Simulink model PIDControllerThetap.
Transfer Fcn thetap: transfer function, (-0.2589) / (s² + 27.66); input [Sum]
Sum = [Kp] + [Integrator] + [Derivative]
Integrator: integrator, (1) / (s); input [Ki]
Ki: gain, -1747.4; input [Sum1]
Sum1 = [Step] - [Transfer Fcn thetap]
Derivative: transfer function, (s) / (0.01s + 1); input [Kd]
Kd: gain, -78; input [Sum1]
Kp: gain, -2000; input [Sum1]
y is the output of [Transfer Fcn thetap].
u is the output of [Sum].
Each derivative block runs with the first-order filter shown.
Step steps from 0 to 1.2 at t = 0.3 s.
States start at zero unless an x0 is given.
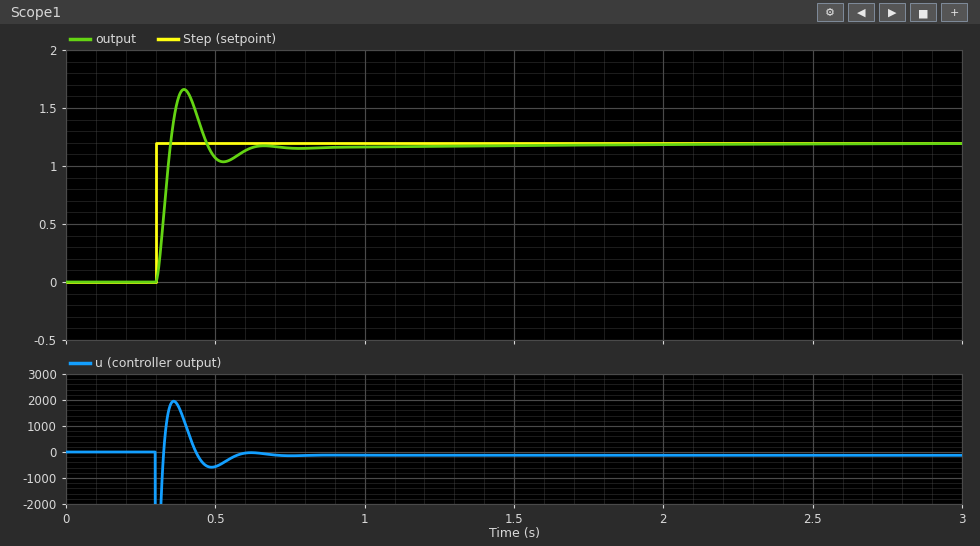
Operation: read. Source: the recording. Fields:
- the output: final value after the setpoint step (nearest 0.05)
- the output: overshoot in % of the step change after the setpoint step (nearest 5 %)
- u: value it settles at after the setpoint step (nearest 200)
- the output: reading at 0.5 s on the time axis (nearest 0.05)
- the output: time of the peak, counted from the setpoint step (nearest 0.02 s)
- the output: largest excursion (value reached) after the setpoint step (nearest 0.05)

1.20
40 %
-200
1.05
0.10 s
1.65
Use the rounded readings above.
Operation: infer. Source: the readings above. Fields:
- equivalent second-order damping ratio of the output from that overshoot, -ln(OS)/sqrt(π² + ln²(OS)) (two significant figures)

0.28
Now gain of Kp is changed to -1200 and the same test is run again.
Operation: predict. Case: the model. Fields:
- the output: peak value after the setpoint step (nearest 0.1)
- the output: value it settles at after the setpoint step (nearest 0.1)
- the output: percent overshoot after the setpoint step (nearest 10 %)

1.5
1.2
30 %
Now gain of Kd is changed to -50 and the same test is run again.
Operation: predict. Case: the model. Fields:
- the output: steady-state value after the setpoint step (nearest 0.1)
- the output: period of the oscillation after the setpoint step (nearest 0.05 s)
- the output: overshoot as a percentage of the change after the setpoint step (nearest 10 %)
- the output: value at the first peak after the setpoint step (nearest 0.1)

1.2
0.25 s
50 %
1.8
